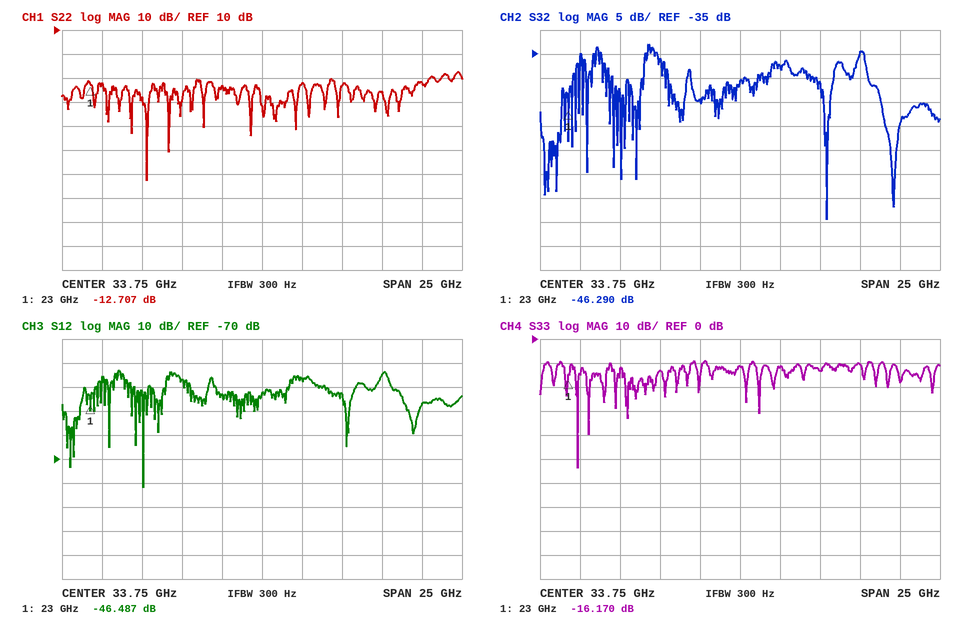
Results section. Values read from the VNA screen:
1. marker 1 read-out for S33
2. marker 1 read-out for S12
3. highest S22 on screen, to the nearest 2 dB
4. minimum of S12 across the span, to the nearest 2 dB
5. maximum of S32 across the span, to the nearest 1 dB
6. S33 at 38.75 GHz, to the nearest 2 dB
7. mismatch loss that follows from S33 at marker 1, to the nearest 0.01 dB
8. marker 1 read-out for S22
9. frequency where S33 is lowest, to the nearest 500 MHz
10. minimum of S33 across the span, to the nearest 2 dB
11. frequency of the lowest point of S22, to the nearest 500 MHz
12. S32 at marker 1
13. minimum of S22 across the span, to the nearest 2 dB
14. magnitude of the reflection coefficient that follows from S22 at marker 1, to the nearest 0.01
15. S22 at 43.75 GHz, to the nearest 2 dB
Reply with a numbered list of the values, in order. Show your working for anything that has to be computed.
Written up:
1. -16.170 dB
2. -46.487 dB
3. -8 dB
4. -82 dB
5. -33 dB
6. -14 dB
7. −10 log10(1 − 10^(-16.17/10)) ≈ 0.11 dB
8. -12.707 dB
9. 23.5 GHz
10. -54 dB
11. 26.5 GHz
12. -46.290 dB
13. -52 dB
14. 10^(-12.707/20) ≈ 0.23
15. -12 dB
